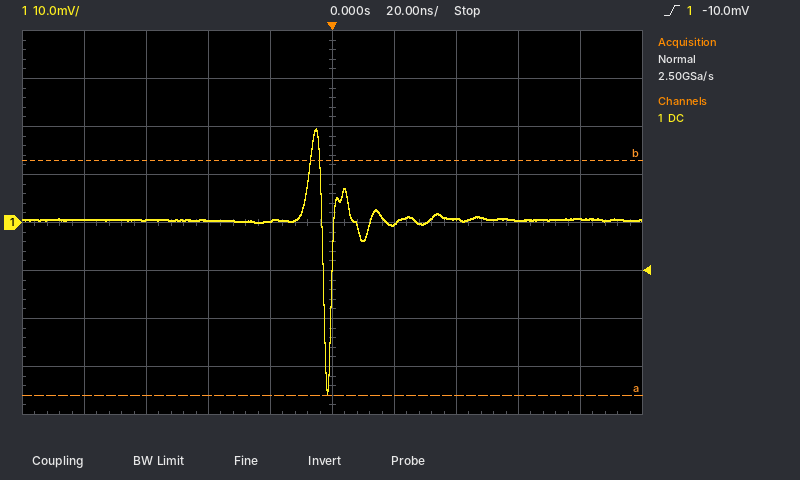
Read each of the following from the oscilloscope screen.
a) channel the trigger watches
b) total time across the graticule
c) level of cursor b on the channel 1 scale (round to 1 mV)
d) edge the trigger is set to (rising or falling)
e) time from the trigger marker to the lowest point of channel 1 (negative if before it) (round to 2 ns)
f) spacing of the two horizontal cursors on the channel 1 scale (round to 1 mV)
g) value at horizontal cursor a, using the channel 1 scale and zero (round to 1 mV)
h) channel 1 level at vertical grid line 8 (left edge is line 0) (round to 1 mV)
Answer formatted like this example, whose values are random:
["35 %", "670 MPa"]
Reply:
["channel 1", "200 ns", "13 mV", "rising", "-2 ns", "49 mV", "-36 mV", "0 mV"]
